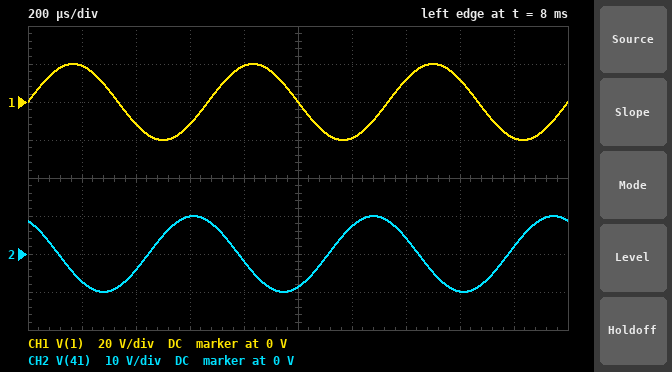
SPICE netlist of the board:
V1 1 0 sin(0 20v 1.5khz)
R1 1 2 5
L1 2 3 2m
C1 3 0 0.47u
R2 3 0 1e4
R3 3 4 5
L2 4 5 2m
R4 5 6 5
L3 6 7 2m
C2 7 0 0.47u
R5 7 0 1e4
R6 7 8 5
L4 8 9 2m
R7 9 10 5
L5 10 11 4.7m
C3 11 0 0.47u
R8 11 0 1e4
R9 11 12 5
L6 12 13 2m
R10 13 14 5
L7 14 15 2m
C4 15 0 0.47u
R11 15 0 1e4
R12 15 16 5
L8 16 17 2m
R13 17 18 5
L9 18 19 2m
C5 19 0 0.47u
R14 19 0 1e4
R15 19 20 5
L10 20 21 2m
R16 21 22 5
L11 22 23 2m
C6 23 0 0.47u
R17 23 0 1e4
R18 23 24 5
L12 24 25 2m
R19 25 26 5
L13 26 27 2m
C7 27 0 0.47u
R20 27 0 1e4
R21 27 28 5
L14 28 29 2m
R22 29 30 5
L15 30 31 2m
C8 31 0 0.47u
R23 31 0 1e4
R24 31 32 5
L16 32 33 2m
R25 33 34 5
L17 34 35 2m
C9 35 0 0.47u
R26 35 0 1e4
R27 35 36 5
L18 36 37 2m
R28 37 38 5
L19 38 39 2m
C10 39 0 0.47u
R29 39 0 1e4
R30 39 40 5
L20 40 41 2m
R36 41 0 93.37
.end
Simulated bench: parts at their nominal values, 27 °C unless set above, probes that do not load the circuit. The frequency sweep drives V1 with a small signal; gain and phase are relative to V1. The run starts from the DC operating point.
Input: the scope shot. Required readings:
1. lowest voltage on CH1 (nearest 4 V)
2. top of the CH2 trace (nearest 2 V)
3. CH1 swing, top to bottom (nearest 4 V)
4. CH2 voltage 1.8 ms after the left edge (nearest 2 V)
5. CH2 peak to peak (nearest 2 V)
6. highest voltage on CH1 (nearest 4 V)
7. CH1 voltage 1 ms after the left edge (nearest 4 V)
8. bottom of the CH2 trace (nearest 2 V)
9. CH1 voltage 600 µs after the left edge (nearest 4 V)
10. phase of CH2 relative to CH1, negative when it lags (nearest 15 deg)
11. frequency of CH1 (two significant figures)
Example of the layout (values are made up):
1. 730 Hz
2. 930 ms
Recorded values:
1. -20 V
2. 10 V
3. 40 V
4. 2 V
5. 20 V
6. 20 V
7. 0 V
8. -10 V
9. -12 V
10. 120 deg
11. 1.5 kHz
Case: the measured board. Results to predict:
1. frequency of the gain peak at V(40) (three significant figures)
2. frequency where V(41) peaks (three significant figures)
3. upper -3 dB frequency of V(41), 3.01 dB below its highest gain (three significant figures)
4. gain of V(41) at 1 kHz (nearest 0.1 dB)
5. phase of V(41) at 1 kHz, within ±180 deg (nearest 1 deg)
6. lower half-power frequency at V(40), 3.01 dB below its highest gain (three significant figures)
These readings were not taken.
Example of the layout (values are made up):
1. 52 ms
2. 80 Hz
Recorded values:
1. 3.81 kHz
2. 3.79 kHz
3. 4.60 kHz
4. -5.4 dB
5. -163 deg
6. 2.70 kHz
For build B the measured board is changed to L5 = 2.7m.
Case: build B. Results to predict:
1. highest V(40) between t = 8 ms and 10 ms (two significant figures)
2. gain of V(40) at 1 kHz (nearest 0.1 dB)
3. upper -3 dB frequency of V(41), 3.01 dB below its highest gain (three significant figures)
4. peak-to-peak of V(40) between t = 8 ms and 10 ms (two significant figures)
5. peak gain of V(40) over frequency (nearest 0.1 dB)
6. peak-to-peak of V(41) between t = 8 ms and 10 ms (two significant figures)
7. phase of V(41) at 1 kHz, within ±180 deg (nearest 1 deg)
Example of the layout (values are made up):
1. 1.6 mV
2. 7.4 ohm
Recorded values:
1. 11 V
2. -5.0 dB
3. 5.67 kHz
4. 22 V
5. -3.4 dB
6. 21 V
7. -157 deg
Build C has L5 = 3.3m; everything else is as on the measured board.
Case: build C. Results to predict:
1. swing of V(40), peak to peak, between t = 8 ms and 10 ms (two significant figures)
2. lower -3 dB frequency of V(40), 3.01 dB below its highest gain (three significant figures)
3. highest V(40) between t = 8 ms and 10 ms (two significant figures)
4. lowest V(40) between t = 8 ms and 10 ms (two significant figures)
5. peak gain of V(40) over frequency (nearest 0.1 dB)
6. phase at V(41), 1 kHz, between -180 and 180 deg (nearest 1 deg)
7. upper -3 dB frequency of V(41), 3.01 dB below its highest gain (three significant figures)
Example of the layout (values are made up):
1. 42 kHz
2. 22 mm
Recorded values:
1. 21 V
2. 389 Hz
3. 11 V
4. -11 V
5. -2.8 dB
6. -159 deg
7. 5.09 kHz
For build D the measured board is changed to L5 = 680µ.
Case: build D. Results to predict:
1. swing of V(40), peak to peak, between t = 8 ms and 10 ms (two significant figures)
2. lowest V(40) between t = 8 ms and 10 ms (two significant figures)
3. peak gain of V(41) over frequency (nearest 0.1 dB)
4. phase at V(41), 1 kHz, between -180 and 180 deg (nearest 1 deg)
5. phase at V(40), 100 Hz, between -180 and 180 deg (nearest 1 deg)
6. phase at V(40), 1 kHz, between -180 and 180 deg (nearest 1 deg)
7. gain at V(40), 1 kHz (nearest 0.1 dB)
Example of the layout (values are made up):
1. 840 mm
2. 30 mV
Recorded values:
1. 23 V
2. -12 V
3. -4.5 dB
4. -151 deg
5. -12 deg
6. -144 deg
7. -4.7 dB
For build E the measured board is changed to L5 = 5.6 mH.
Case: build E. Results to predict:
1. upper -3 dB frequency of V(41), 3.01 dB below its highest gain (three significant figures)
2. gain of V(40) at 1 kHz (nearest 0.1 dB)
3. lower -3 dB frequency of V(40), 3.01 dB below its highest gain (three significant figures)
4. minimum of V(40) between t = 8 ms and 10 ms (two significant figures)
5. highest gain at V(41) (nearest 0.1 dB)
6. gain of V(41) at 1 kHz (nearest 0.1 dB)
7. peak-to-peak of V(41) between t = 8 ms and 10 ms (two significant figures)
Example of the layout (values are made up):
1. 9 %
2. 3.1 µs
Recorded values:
1. 4.38 kHz
2. -5.5 dB
3. 2.86 kHz
4. -9.8 V
5. -2.2 dB
6. -5.6 dB
7. 19 V
